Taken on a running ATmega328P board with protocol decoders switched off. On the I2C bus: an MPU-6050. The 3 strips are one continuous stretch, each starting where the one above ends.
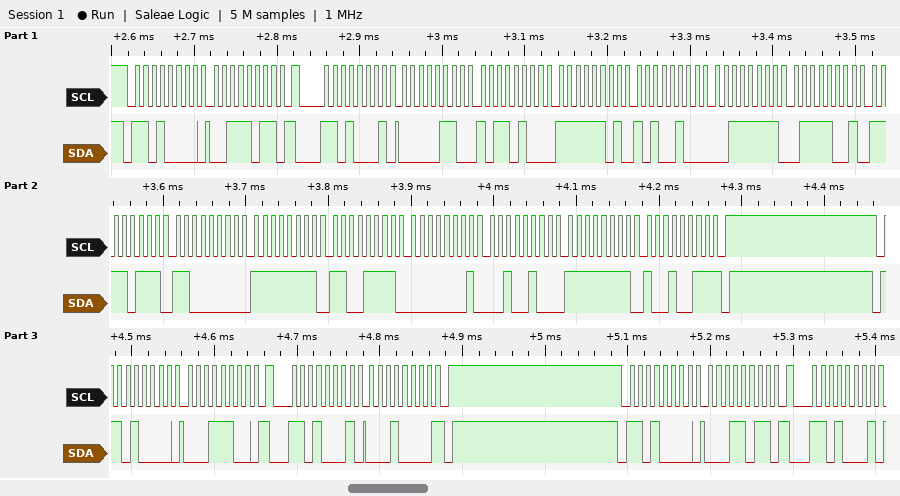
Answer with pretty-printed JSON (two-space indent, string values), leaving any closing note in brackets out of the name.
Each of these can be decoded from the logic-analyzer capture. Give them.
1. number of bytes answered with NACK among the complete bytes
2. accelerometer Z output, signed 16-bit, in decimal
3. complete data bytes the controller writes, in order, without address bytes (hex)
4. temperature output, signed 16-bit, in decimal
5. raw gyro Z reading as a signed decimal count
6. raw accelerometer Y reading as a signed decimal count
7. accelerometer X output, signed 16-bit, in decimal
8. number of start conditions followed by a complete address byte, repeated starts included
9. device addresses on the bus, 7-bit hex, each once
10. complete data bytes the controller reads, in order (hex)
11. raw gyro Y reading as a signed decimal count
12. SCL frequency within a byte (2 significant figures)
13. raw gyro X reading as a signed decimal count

{
  "number of bytes answered with NACK among the complete bytes": "2",
  "accelerometer Z output, signed 16-bit, in decimal": "16249",
  "complete data bytes the controller writes, in order, without address bytes": "3B 1C 1B",
  "temperature output, signed 16-bit, in decimal": "-2112",
  "raw gyro Z reading as a signed decimal count": "-109",
  "raw accelerometer Y reading as a signed decimal count": "-604",
  "accelerometer X output, signed 16-bit, in decimal": "1716",
  "number of start conditions followed by a complete address byte, repeated starts included": "6",
  "device addresses on the bus, 7-bit hex, each once": "0x68",
  "complete data bytes the controller reads, in order": "06 B4 FD A4 3F 79 F7 C0 FF CF 01 24 FF 93 10",
  "raw gyro Y reading as a signed decimal count": "292",
  "SCL frequency within a byte": "100 kHz",
  "raw gyro X reading as a signed decimal count": "-49"
}
